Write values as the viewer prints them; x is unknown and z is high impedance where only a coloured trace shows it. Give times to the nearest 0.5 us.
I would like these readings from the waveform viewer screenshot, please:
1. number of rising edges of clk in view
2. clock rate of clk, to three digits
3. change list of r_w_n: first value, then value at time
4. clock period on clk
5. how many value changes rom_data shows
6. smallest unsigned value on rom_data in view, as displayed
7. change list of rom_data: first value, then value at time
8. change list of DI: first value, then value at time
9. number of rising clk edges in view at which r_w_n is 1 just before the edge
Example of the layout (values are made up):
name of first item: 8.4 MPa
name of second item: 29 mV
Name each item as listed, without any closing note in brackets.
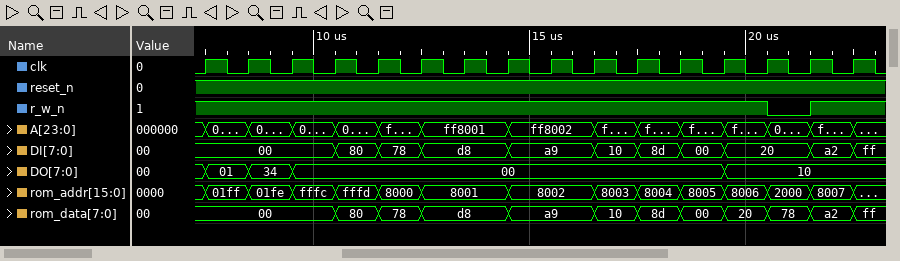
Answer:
number of rising edges of clk in view: 16
clock rate of clk, to three digits: 1.00 MHz
change list of r_w_n: first value, then value at time: 1, 0 at 20.5 us, 1 at 21.5 us
clock period on clk: 1 us
how many value changes rom_data shows: 11
smallest unsigned value on rom_data in view, as displayed: 00
change list of rom_data: first value, then value at time: 00, 80 at 10.5 us, 78 at 11.5 us, d8 at 12.5 us, a9 at 14.5 us, 10 at 16.5 us, 8d at 17.5 us, 00 at 18.5 us, 20 at 19.5 us, 78 at 20.5 us, a2 at 21.5 us, ff at 22.5 us
change list of DI: first value, then value at time: 00, 80 at 10.5 us, 78 at 11.5 us, d8 at 12.5 us, a9 at 14.5 us, 10 at 16.5 us, 8d at 17.5 us, 00 at 18.5 us, 20 at 19.5 us, a2 at 21.5 us, ff at 22.5 us
number of rising clk edges in view at which r_w_n is 1 just before the edge: 15
